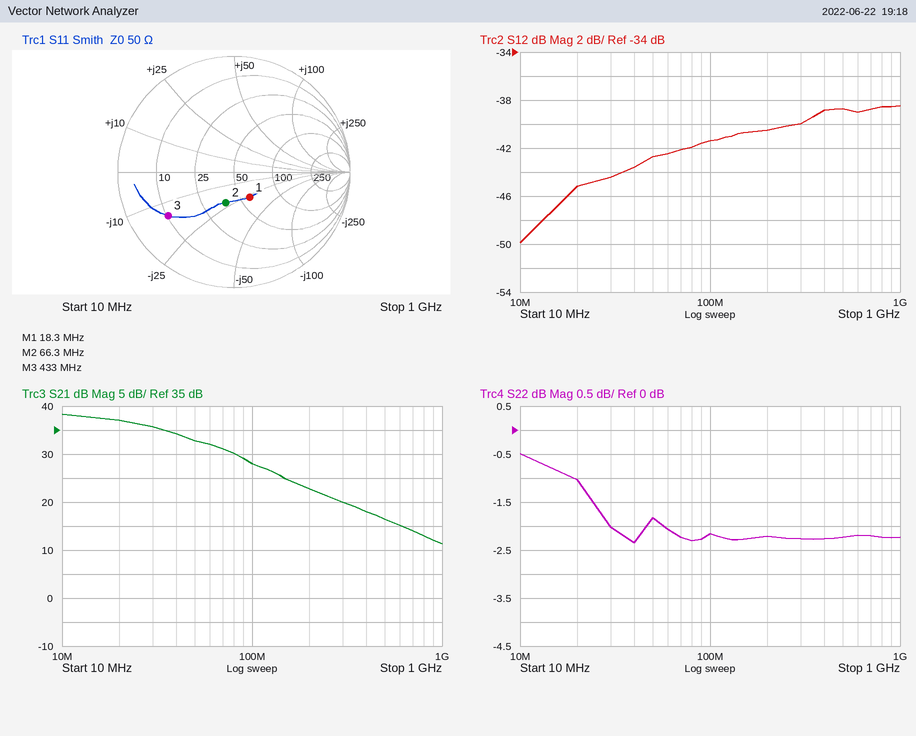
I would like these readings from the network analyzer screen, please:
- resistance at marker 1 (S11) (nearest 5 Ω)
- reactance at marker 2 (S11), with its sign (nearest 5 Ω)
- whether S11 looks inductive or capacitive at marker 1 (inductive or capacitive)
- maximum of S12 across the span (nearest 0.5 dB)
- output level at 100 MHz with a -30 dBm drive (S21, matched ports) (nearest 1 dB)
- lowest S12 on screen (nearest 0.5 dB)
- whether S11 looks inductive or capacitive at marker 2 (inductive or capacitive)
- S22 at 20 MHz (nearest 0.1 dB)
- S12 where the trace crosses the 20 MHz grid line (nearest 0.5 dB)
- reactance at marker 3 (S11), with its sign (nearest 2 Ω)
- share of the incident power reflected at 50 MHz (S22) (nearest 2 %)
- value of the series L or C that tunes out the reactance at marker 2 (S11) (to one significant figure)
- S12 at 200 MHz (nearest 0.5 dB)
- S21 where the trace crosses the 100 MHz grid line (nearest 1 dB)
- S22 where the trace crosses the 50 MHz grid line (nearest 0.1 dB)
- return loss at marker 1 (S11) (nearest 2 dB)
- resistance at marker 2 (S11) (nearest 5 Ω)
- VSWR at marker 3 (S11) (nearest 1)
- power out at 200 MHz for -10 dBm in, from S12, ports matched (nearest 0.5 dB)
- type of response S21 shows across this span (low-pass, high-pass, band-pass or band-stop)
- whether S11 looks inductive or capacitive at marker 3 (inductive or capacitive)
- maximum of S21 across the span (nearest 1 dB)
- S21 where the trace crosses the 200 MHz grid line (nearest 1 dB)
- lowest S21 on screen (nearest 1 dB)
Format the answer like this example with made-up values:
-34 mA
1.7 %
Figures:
60 Ω
-20 Ω
capacitive
-38.5 dB
-2 dBm
-50.0 dB
capacitive
-1.0 dB
-45.0 dB
-14 Ω
66 %
50 nH
-40.5 dB
28 dB
-1.8 dB
12 dB
40 Ω
5
-50.5 dBm
low-pass
capacitive
38 dB
23 dB
11 dB
